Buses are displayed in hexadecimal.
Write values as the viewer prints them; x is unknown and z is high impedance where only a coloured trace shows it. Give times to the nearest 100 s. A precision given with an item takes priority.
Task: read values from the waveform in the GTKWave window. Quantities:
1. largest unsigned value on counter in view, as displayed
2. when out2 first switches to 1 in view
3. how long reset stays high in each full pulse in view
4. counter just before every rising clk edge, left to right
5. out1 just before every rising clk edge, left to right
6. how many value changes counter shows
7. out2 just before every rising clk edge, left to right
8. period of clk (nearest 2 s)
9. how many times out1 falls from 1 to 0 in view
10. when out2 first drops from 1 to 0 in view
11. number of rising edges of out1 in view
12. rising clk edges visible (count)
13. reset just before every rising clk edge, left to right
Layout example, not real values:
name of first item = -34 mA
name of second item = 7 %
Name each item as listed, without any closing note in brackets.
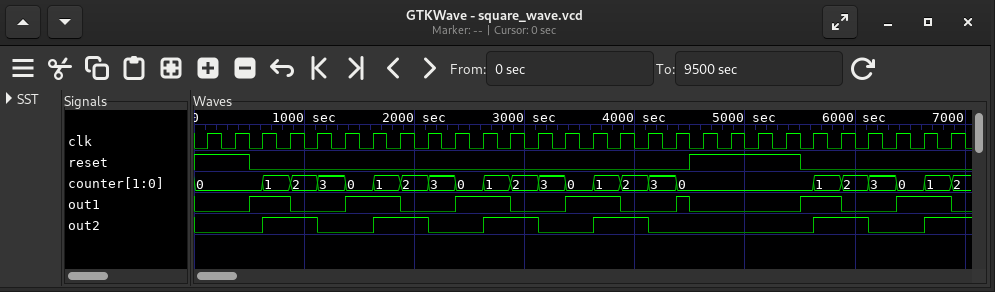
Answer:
largest unsigned value on counter in view, as displayed = 3
when out2 first switches to 1 in view = 600 s
how long reset stays high in each full pulse in view = 1000 s
counter just before every rising clk edge, left to right = 0, 0, 0, 1, 2, 3, 0, 1, 2, 3, 0, 1, 2, 3, 0, 1, 2, 3, 0, 0, 0, 0, 0, 1, 2, 3, 0, 1
out1 just before every rising clk edge, left to right = 0 0 1 1 0 0 1 1 0 0 1 1 0 0 1 1 0 0 0 0 0 0 1 1 0 0 1 1
how many value changes counter shows = 22
out2 just before every rising clk edge, left to right = 0 0 0 1 1 0 0 1 1 0 0 1 1 0 0 1 1 0 0 0 0 0 0 1 1 0 0 1
period of clk = 250 s
how many times out1 falls from 1 to 0 in view = 7
when out2 first drops from 1 to 0 in view = 1100 s
number of rising edges of out1 in view = 7
rising clk edges visible = 28
reset just before every rising clk edge, left to right = 1 1 0 0 0 0 0 0 0 0 0 0 0 0 0 0 0 0 1 1 1 1 0 0 0 0 0 0
